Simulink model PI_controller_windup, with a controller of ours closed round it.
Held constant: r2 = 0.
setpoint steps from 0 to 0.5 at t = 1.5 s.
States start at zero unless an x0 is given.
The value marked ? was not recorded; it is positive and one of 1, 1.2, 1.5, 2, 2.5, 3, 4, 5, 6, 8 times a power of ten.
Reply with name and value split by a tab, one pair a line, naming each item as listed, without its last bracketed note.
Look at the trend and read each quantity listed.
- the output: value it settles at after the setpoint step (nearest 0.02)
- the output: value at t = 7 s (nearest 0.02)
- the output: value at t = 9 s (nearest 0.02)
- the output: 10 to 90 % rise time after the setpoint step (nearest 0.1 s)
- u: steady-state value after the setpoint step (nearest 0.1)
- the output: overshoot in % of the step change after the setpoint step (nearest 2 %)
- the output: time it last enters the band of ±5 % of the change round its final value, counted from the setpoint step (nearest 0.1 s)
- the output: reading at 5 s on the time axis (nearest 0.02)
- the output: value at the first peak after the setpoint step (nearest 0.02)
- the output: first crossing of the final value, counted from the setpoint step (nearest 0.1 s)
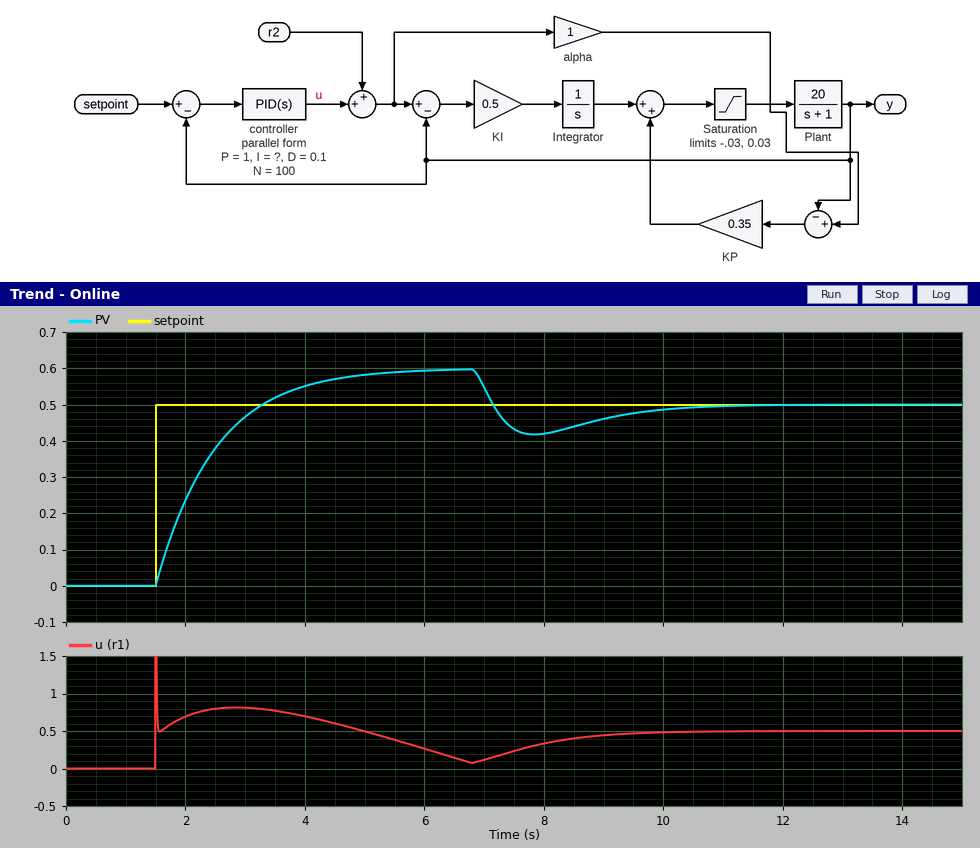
the output: value it settles at after the setpoint step	0.50
the output: value at t = 7 s	0.54
the output: value at t = 9 s	0.46
the output: 10 to 90 % rise time after the setpoint step	1.3 s
u: steady-state value after the setpoint step	0.5
the output: overshoot in % of the step change after the setpoint step	20 %
the output: time it last enters the band of ±5 % of the change round its final value, counted from the setpoint step	8.0 s
the output: reading at 5 s on the time axis	0.58
the output: value at the first peak after the setpoint step	0.60
the output: first crossing of the final value, counted from the setpoint step	1.8 s
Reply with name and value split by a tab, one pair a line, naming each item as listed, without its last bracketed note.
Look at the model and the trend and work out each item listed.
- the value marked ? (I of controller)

the value marked ?	2.5
